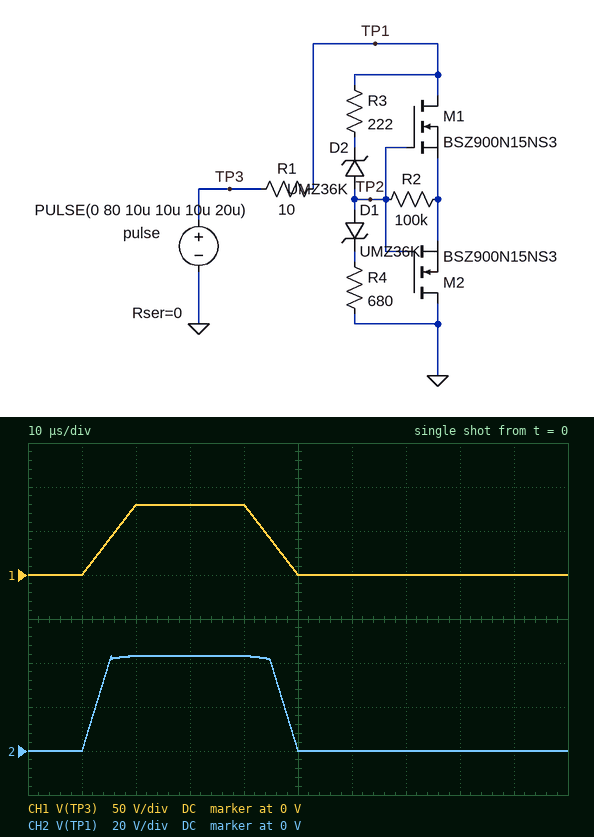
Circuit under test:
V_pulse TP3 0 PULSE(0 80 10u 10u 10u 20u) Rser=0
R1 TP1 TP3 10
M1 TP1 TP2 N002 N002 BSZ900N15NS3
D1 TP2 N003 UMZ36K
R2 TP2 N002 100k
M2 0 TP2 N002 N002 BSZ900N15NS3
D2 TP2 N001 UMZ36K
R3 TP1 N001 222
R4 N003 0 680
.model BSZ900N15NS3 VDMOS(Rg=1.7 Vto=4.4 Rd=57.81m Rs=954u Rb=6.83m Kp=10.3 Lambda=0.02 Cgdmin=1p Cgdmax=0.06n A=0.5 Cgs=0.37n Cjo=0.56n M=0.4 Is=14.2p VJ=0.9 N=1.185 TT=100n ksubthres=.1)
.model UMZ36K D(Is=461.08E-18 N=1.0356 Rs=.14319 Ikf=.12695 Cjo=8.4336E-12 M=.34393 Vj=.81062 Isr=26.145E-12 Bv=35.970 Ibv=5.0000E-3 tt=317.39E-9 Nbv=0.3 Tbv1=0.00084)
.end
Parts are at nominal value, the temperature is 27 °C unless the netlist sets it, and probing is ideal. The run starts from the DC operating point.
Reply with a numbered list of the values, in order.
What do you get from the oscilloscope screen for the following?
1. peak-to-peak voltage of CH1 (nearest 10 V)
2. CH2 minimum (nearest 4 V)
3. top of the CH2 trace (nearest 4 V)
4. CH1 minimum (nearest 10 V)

1. 80 V
2. 0 V
3. 44 V
4. 0 V
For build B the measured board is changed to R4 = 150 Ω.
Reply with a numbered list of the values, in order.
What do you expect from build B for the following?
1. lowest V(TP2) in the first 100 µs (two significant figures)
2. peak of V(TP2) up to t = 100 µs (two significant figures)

1. -15 V
2. 5.5 V
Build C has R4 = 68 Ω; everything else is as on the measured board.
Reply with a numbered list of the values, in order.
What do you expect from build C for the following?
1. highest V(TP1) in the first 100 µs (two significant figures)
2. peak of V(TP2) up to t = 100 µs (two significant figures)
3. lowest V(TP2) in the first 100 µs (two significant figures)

1. 56 V
2. 5.4 V
3. -15 V
